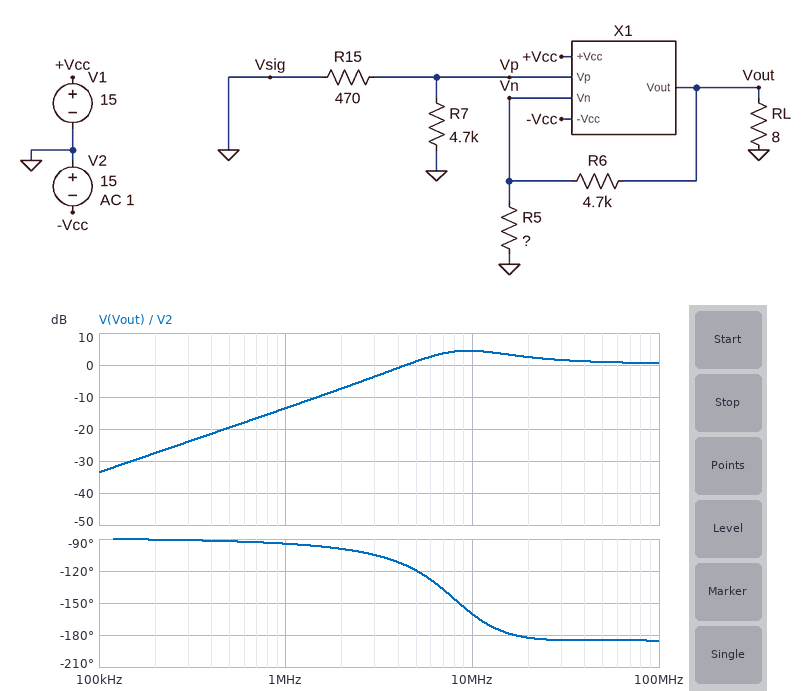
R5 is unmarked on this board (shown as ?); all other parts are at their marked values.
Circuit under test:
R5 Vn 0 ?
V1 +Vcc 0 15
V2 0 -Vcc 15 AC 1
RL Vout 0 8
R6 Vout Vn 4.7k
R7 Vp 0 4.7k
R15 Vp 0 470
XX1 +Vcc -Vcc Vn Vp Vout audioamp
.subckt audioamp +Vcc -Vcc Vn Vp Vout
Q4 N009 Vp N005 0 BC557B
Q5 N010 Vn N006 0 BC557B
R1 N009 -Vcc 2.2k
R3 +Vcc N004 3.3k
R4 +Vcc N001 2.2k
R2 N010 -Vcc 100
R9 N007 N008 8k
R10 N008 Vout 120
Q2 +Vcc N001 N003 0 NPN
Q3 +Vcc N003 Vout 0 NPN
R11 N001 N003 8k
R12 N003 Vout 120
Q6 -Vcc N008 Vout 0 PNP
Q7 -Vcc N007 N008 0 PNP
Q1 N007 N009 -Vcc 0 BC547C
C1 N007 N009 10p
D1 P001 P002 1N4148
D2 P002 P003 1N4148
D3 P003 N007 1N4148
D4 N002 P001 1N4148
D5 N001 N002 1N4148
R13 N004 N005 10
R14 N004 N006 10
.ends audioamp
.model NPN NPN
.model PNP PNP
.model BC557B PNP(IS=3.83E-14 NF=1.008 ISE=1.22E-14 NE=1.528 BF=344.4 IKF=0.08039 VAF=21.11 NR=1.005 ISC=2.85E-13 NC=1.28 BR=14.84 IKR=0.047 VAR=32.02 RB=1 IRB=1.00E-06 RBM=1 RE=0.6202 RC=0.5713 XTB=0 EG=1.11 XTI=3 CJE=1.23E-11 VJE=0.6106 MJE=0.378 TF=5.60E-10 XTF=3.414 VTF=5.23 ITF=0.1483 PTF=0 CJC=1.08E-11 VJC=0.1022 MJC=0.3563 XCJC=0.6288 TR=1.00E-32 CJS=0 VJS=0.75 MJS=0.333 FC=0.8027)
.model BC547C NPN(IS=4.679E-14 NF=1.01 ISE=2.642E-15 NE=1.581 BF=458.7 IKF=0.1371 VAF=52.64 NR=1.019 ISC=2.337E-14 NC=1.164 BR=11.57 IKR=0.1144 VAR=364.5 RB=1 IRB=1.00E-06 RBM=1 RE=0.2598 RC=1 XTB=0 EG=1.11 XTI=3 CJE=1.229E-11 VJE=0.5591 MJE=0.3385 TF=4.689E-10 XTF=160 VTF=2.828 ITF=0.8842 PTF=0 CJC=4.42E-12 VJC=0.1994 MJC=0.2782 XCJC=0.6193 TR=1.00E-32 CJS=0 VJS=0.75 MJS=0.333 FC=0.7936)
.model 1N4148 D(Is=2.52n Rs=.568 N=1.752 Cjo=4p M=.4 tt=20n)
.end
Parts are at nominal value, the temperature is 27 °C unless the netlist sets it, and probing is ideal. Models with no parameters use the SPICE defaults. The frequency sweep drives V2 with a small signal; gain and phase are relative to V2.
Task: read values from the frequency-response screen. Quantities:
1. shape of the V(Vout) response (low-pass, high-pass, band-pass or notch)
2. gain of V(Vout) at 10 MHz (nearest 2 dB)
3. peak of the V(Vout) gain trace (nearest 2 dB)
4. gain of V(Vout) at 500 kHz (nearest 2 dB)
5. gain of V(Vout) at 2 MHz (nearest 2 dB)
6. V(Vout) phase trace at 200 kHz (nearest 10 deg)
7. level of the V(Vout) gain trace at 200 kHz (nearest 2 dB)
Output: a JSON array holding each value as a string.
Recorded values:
["high-pass", "4 dB", "4 dB", "-20 dB", "-8 dB", "-90 deg", "-28 dB"]
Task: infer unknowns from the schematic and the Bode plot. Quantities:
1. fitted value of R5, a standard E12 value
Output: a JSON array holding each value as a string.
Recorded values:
["270 Ω"]
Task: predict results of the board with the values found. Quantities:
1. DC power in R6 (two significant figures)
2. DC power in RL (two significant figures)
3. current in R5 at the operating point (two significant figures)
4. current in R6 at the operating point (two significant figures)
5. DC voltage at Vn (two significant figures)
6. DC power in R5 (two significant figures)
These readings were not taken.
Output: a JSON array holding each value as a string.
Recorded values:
["760 µW", "500 mW", "390 µA", "400 µA", "-110 mV", "42 µW"]
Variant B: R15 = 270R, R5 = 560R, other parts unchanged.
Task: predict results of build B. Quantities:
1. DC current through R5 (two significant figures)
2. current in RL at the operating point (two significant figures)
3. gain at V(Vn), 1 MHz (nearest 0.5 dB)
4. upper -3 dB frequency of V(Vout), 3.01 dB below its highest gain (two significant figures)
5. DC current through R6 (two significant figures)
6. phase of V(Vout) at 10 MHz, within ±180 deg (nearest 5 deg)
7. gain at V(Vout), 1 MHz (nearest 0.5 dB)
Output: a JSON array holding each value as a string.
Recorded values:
["190 µA", "130 mA", "-38.0 dB", "51 MHz", "200 µA", "-105 deg", "-24.0 dB"]
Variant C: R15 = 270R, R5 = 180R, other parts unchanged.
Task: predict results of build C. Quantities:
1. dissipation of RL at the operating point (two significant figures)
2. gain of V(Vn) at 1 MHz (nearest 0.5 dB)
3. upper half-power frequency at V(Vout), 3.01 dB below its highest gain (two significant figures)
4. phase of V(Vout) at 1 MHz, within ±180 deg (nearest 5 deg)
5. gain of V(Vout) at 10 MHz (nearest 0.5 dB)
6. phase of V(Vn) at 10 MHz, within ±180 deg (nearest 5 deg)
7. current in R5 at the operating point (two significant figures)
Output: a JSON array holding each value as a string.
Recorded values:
["1.1 W", "-38.5 dB", "250 MHz", "-100 deg", "3.0 dB", "-145 deg", "590 µA"]
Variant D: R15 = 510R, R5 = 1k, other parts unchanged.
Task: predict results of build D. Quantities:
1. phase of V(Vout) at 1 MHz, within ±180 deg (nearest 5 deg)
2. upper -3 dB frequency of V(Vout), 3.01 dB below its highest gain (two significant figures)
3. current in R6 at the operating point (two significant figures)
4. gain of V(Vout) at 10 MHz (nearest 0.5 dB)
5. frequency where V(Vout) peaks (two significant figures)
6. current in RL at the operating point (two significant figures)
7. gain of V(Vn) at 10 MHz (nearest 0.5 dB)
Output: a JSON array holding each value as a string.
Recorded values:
["-75 deg", "18 MHz", "110 µA", "4.0 dB", "13 MHz", "80 mA", "-10.0 dB"]
